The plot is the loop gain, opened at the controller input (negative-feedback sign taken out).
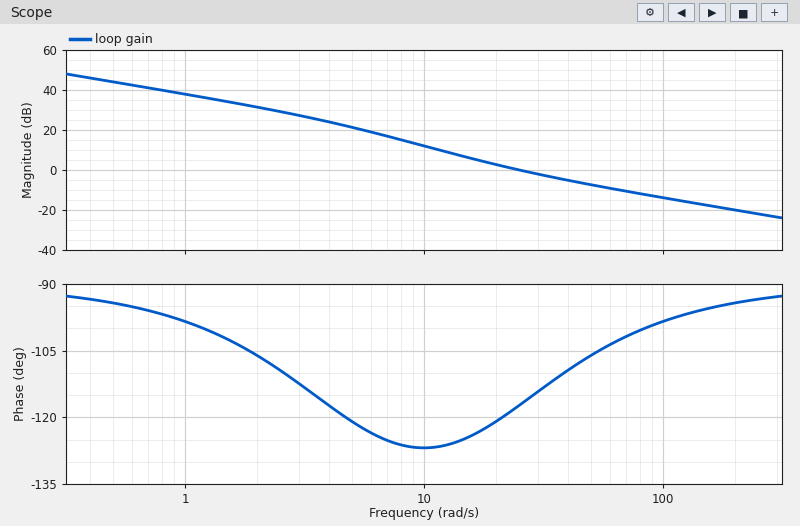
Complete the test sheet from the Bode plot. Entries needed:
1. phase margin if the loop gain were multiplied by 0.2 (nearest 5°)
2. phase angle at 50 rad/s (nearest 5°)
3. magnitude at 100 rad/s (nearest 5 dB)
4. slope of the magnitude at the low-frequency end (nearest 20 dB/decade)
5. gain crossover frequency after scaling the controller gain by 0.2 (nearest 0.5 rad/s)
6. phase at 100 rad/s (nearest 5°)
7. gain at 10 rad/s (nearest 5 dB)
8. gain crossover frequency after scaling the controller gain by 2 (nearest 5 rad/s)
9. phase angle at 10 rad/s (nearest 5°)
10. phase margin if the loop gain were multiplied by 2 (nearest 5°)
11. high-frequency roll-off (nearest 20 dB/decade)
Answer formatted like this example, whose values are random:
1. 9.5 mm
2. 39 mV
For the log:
1. 55°
2. -105°
3. -15 dB
4. -20 dB/decade
5. 8.5 rad/s
6. -100°
7. 10 dB
8. 45 rad/s
9. -125°
10. 70°
11. -20 dB/decade
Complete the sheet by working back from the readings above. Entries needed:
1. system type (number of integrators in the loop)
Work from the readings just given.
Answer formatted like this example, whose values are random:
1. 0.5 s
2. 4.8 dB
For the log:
1. 1
